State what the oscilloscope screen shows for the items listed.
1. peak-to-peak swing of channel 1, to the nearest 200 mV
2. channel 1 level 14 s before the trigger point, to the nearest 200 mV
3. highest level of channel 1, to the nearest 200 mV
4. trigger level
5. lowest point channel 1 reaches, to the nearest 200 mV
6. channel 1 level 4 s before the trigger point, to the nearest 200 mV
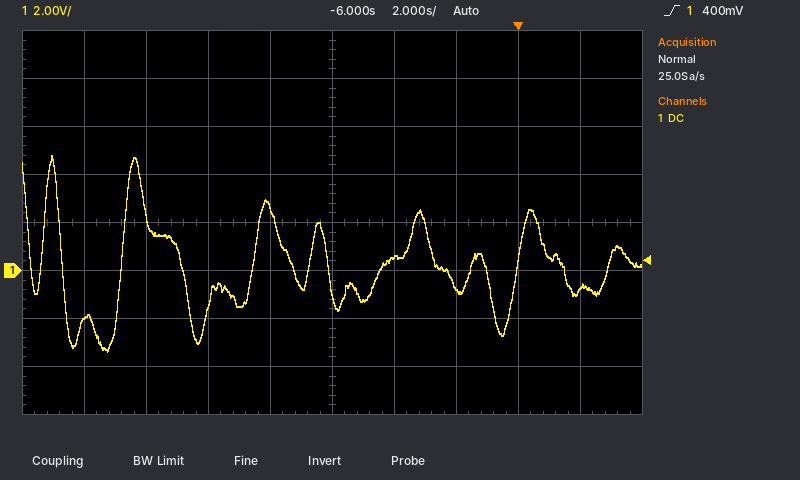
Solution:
8.2 V
-2.0 V
4.8 V
400 mV
-3.4 V
600 mV
